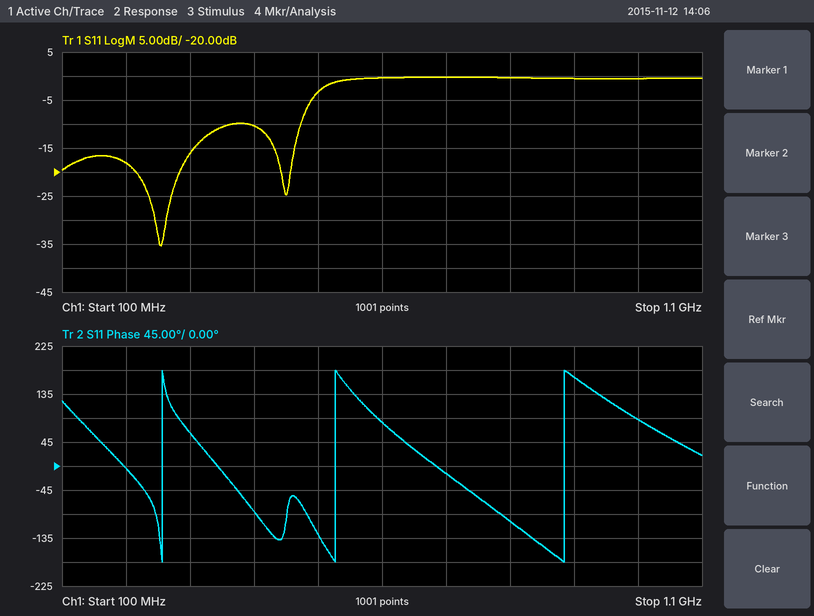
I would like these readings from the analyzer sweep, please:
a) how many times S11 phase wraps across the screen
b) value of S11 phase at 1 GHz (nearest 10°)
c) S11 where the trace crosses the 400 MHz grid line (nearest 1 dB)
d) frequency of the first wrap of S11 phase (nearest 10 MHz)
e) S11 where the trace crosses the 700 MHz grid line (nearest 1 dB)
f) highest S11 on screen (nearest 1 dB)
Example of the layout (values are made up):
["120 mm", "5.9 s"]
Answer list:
["3", "90°", "-10 dB", "260 MHz", "0 dB", "0 dB"]
